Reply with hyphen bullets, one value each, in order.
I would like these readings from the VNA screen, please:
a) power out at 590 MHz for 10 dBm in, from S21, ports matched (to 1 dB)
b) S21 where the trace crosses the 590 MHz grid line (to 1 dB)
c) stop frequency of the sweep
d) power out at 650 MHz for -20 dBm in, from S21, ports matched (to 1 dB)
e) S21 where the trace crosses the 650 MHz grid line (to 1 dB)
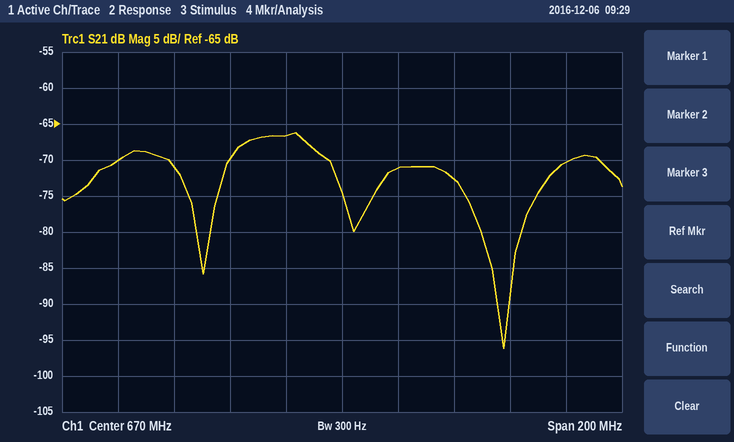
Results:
- -60 dBm
- -70 dB
- 770 MHz
- -87 dBm
- -67 dB
